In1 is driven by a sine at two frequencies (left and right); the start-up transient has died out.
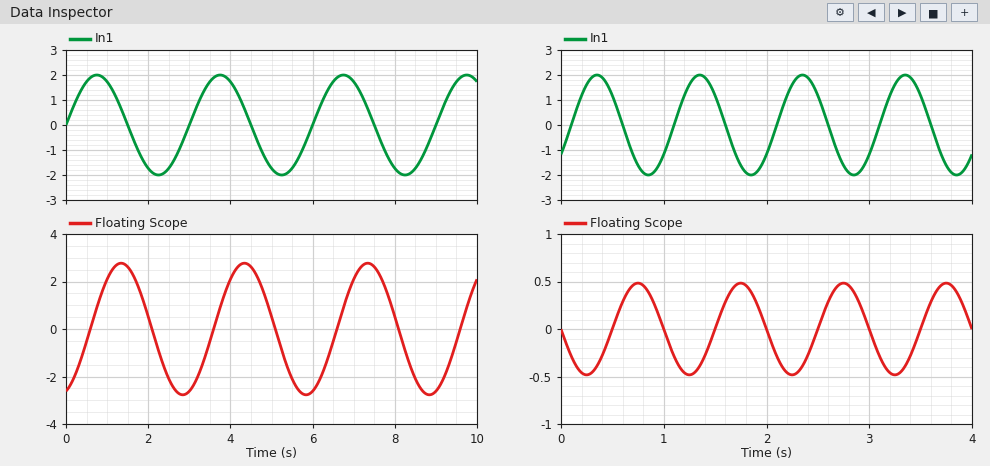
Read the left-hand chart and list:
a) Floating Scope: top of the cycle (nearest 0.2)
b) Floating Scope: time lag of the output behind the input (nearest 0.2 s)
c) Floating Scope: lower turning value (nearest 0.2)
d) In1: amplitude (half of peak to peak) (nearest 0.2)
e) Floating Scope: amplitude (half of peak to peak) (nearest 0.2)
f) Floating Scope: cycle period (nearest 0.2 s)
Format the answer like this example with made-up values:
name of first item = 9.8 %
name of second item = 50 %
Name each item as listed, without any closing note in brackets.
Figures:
Floating Scope: top of the cycle = 2.8
Floating Scope: time lag of the output behind the input = 0.6 s
Floating Scope: lower turning value = -2.8
In1: amplitude (half of peak to peak) = 2.0
Floating Scope: amplitude (half of peak to peak) = 2.8
Floating Scope: cycle period = 3.0 s
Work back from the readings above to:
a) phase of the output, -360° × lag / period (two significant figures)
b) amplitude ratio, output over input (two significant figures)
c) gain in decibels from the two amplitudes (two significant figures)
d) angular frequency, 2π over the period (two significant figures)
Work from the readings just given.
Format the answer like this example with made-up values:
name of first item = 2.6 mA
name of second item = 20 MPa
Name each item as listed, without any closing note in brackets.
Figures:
phase of the output, -360° × lag / period = -72°
amplitude ratio, output over input = 1.4
gain in decibels from the two amplitudes = 2.9 dB
angular frequency, 2π over the period = 2.1 rad/s
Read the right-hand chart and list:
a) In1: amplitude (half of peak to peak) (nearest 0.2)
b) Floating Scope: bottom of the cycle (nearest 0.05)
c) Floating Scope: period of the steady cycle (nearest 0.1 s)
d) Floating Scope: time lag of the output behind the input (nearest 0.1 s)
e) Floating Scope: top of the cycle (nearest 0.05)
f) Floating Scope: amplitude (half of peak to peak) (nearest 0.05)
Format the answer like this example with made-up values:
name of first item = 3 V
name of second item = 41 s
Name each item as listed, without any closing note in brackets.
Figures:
In1: amplitude (half of peak to peak) = 2.0
Floating Scope: bottom of the cycle = -0.50
Floating Scope: period of the steady cycle = 1.0 s
Floating Scope: time lag of the output behind the input = 0.4 s
Floating Scope: top of the cycle = 0.50
Floating Scope: amplitude (half of peak to peak) = 0.50
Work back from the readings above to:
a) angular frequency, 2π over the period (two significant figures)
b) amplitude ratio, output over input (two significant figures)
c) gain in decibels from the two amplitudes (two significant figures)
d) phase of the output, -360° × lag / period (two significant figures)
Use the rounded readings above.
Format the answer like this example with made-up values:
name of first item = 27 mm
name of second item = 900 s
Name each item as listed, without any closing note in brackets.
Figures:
angular frequency, 2π over the period = 6.3 rad/s
amplitude ratio, output over input = 0.25
gain in decibels from the two amplitudes = -12 dB
phase of the output, -360° × lag / period = -140°
